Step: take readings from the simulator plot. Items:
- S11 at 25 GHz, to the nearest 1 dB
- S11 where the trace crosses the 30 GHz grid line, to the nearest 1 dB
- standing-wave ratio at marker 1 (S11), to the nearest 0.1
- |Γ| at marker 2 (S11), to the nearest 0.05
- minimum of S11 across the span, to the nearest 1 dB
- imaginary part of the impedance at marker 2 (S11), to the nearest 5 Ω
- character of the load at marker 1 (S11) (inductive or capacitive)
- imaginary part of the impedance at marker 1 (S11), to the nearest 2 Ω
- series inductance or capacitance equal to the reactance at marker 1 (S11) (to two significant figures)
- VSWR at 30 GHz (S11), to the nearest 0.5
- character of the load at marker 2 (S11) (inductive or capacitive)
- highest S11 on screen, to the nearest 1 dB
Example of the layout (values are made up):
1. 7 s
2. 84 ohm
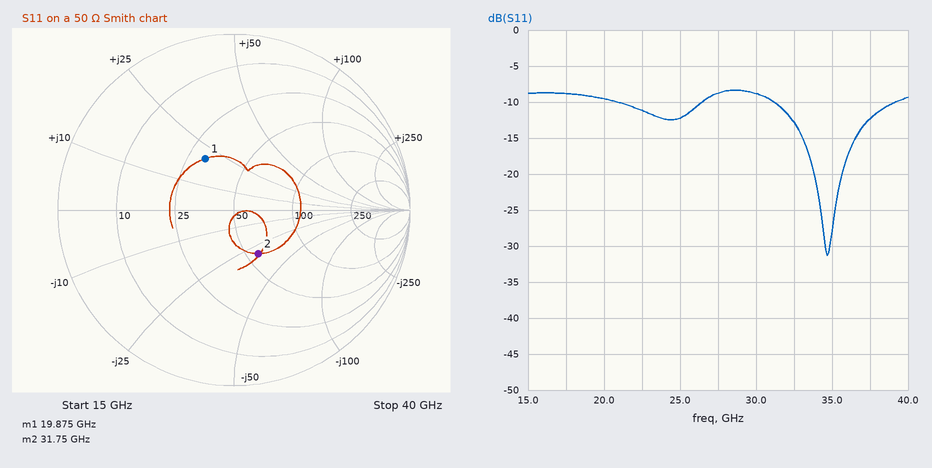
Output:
1. -12 dB
2. -9 dB
3. 2.0
4. 0.30
5. -31 dB
6. -30 Ω
7. inductive
8. +20 Ω
9. 160 pH
10. 2.0
11. capacitive
12. -8 dB
